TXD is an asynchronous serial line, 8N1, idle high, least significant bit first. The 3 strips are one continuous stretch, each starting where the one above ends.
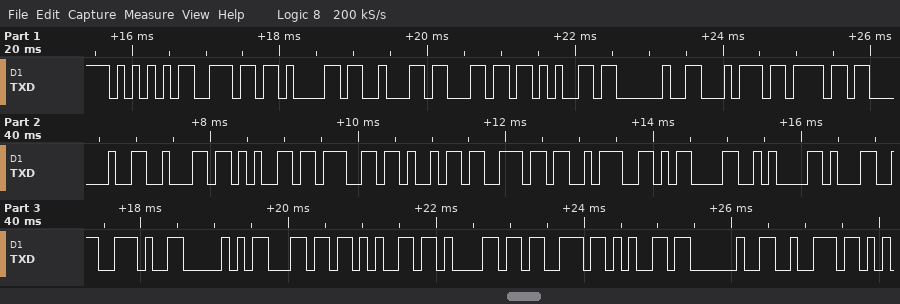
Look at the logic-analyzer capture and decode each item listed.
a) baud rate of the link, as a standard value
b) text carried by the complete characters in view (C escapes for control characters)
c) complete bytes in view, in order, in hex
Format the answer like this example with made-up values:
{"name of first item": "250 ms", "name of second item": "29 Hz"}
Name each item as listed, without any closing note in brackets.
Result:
{"baud rate of the link, as a standard value": "9600 baud", "text carried by the complete characters in view": "\"Unable to begin:\\r\\n1.Please r\"", "complete bytes in view, in order, in hex": "55 6E 61 62 6C 65 20 74 6F 20 62 65 67 69 6E 3A 0D 0A 31 2E 50 6C 65 61 73 65 20 72"}
